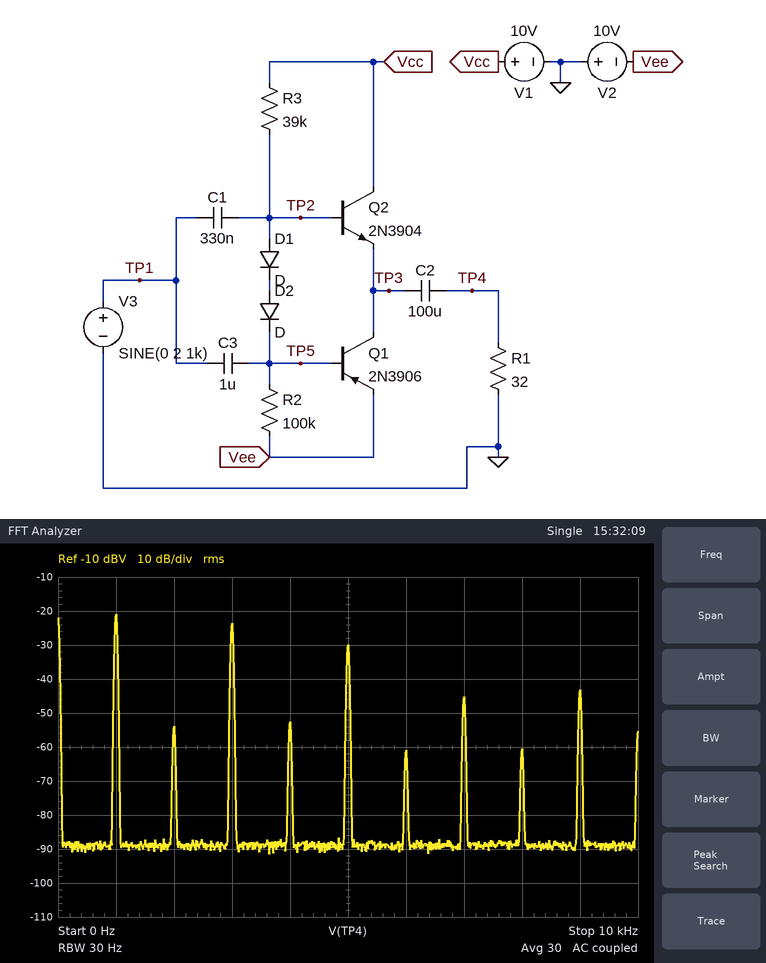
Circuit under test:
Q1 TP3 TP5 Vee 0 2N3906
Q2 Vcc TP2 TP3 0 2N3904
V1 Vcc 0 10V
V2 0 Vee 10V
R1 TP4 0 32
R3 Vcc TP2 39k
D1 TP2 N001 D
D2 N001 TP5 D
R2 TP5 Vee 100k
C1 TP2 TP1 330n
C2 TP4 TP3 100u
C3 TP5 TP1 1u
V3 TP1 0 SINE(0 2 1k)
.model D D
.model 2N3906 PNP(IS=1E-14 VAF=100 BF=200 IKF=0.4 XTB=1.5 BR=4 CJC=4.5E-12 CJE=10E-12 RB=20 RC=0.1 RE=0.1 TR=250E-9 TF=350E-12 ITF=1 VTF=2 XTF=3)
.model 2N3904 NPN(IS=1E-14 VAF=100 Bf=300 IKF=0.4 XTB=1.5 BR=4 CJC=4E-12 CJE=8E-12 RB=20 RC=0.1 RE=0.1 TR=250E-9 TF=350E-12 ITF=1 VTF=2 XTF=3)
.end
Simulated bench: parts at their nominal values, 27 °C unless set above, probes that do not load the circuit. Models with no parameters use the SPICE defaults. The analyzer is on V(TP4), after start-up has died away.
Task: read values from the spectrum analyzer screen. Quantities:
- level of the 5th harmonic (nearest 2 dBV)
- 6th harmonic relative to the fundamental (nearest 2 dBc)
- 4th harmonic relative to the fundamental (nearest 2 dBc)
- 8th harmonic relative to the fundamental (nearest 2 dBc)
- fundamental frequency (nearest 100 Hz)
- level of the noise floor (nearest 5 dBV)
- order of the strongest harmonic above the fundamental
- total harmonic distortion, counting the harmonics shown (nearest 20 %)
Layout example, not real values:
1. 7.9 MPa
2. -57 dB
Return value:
1. -30 dBV
2. -40 dBc
3. -32 dBc
4. -40 dBc
5. 1.0 kHz
6. -90 dBV
7. 3
8. 80 %
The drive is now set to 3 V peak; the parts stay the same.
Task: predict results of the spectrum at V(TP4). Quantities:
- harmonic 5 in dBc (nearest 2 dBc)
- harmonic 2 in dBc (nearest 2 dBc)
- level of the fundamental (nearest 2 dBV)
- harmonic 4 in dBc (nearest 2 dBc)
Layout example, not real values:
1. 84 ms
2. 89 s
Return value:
1. -6 dBc
2. -42 dBc
3. -20 dBV
4. -36 dBc
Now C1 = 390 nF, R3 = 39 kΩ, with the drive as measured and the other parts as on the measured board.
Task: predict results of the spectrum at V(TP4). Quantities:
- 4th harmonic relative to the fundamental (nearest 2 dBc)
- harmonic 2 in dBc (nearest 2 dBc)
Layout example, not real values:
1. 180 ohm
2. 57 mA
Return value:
1. -28 dBc
2. -30 dBc
